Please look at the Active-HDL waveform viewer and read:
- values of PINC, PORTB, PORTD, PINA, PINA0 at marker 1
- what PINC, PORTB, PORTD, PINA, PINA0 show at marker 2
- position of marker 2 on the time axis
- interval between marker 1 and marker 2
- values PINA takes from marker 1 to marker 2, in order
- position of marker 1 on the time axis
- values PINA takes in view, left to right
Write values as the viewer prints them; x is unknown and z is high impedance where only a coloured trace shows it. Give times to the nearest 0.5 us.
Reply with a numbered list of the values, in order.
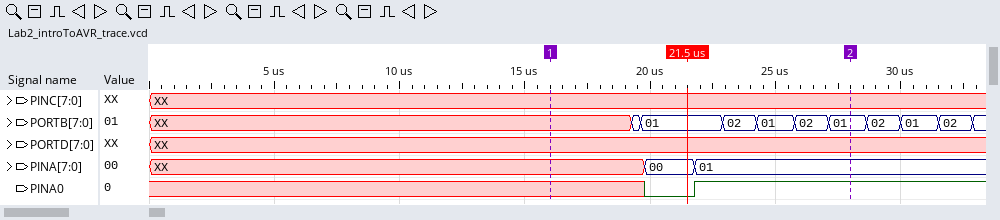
1. PINC=XX, PORTB=XX, PORTD=XX, PINA=XX, PINA0=x
2. PINC=XX, PORTB=01, PORTD=XX, PINA=01, PINA0=1
3. 28 us
4. 12 us
5. XX, 00, 01
6. 16 us
7. XX, 00, 01
